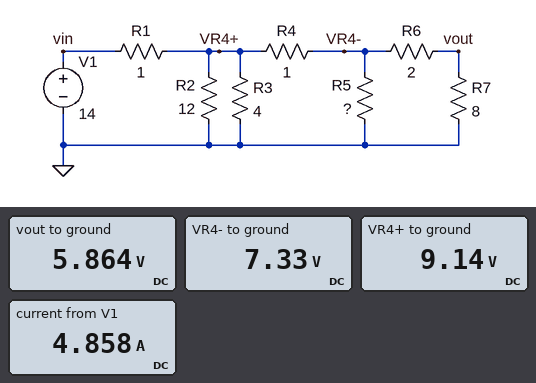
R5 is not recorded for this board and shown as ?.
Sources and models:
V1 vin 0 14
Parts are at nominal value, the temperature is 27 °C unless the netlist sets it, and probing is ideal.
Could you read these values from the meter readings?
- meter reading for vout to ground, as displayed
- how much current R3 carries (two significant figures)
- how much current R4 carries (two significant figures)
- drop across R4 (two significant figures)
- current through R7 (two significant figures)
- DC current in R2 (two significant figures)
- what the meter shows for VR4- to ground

5.864 V
2.3 A
1.8 A
1.8 V
730 mA
760 mA
7.33 V
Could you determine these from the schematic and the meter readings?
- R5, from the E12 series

6.8 Ω
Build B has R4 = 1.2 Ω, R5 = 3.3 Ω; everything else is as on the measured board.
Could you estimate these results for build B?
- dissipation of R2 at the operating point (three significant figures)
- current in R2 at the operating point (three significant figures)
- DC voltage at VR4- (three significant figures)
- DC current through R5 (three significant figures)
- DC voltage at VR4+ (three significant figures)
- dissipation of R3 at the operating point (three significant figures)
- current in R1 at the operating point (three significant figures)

6.34 W
727 mA
5.88 V
1.78 A
8.72 V
19.0 W
5.28 A
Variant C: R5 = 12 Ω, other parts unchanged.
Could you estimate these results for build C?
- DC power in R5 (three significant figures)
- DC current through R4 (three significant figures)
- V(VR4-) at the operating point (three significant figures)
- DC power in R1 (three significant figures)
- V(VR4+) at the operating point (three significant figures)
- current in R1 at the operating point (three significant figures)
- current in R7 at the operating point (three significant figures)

5.27 W
1.46 A
7.95 V
21.1 W
9.41 V
4.59 A
795 mA
